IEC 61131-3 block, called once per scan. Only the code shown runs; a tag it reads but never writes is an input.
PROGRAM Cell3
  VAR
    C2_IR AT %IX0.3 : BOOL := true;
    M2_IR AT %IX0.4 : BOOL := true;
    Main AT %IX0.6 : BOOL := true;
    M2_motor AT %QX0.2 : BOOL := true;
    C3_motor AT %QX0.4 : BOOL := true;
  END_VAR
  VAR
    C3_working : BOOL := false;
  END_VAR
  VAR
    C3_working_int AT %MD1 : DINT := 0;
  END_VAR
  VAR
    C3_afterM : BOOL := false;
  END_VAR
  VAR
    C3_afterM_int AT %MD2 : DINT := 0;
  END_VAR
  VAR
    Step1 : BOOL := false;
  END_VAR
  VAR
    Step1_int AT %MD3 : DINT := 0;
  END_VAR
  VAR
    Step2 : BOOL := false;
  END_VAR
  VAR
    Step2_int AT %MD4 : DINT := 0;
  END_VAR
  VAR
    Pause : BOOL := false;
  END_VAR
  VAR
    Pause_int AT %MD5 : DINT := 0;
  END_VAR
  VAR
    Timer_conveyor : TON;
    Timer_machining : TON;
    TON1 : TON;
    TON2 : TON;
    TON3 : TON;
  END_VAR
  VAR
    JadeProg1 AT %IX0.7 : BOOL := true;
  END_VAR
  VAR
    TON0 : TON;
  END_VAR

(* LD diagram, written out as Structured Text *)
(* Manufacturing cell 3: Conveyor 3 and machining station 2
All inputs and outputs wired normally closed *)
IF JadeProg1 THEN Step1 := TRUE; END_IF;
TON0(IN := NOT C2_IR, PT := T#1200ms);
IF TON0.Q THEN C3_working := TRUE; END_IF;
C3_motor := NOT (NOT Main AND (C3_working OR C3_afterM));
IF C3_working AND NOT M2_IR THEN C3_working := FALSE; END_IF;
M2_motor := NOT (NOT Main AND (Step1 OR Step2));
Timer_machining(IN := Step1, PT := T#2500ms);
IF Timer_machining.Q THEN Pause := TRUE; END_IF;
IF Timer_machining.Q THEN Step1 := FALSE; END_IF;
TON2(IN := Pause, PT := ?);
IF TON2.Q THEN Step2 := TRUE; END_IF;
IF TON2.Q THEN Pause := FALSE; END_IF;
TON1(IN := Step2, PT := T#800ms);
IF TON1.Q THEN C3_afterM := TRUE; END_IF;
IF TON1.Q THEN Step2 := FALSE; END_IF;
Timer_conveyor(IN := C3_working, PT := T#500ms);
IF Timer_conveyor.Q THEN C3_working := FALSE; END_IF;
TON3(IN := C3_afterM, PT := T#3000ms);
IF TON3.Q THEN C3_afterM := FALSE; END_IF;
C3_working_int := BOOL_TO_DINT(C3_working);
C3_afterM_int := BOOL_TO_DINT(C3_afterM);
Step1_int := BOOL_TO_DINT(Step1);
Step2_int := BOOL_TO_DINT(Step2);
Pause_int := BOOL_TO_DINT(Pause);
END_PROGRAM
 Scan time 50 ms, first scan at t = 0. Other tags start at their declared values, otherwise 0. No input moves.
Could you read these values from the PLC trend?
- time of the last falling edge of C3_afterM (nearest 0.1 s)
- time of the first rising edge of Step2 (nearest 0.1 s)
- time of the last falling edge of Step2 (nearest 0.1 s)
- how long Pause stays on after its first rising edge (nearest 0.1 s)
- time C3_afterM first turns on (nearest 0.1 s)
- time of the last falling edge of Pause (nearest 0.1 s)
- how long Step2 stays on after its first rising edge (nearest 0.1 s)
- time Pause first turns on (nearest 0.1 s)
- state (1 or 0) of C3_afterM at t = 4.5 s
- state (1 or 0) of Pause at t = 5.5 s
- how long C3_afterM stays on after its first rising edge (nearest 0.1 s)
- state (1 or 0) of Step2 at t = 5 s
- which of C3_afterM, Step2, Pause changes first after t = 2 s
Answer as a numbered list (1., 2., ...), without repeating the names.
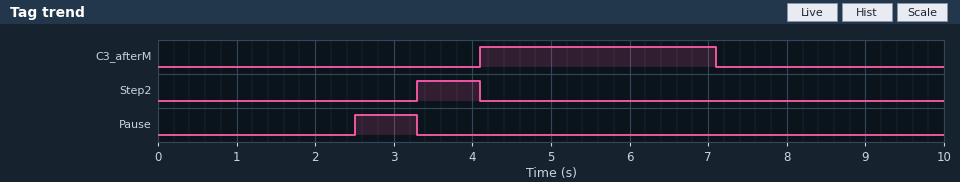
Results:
1. 7.1 s
2. 3.3 s
3. 4.1 s
4. 0.8 s
5. 4.1 s
6. 3.3 s
7. 0.8 s
8. 2.5 s
9. 1
10. 0
11. 3.0 s
12. 0
13. Pause
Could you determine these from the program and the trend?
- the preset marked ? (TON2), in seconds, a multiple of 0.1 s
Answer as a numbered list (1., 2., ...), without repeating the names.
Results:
1. 0.8 s
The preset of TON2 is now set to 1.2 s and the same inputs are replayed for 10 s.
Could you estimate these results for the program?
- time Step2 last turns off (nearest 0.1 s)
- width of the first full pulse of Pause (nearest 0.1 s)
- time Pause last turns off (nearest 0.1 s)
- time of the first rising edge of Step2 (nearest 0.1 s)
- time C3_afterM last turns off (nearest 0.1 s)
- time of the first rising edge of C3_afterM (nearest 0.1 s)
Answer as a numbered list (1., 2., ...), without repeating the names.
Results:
1. 4.5 s
2. 1.2 s
3. 3.7 s
4. 3.7 s
5. 7.5 s
6. 4.5 s
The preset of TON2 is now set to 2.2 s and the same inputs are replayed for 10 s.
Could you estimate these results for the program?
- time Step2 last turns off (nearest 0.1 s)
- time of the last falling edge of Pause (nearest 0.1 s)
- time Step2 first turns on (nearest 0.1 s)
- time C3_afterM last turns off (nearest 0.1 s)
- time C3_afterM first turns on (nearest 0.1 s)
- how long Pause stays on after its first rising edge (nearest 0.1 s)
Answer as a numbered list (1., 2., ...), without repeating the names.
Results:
1. 5.5 s
2. 4.7 s
3. 4.7 s
4. 8.5 s
5. 5.5 s
6. 2.2 s
